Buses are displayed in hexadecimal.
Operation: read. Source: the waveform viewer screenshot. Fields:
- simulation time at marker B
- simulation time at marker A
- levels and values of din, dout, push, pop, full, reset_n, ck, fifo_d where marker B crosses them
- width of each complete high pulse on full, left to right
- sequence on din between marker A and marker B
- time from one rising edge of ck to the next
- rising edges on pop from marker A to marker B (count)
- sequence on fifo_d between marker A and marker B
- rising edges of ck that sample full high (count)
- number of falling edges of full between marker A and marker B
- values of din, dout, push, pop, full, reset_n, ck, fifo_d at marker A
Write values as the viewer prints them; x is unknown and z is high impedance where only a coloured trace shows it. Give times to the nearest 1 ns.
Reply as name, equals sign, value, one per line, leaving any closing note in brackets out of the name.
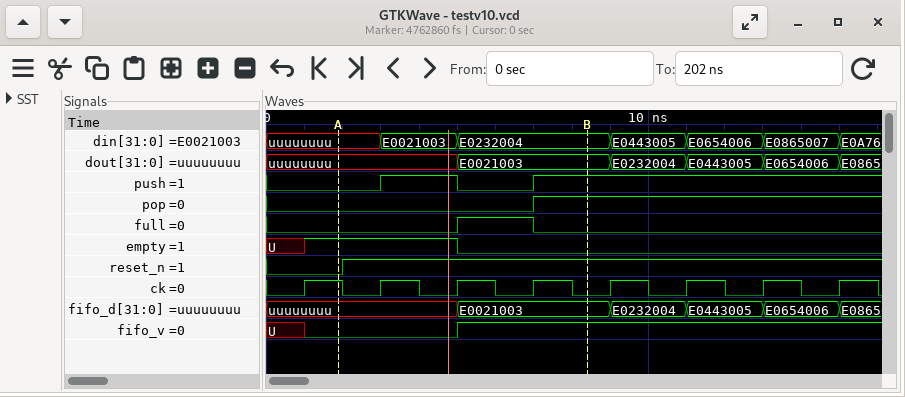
simulation time at marker B = 8 ns
simulation time at marker A = 2 ns
levels and values of din, dout, push, pop, full, reset_n, ck, fifo_d where marker B crosses them = din=E0232004, dout=E0021003, push=1, pop=1, full=0, reset_n=1, ck=0, fifo_d=E0021003
width of each complete high pulse on full, left to right = 2 ns
sequence on din between marker A and marker B = uuuuuuuu, E0021003, E0232004
time from one rising edge of ck to the next = 2 ns
rising edges on pop from marker A to marker B = 1
sequence on fifo_d between marker A and marker B = uuuuuuuu, E0021003
rising edges of ck that sample full high = 1
number of falling edges of full between marker A and marker B = 1
values of din, dout, push, pop, full, reset_n, ck, fifo_d at marker A = din=uuuuuuuu, dout=uuuuuuuu, push=0, pop=0, full=0, reset_n=0, ck=1, fifo_d=uuuuuuuu
